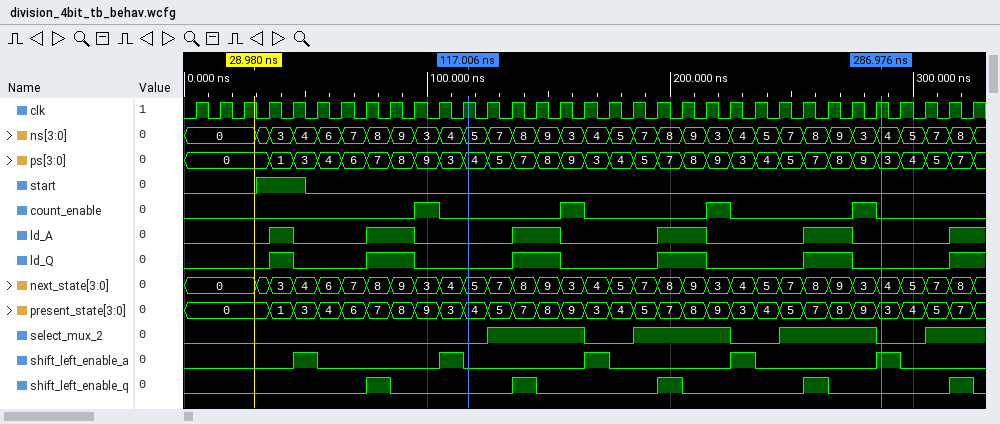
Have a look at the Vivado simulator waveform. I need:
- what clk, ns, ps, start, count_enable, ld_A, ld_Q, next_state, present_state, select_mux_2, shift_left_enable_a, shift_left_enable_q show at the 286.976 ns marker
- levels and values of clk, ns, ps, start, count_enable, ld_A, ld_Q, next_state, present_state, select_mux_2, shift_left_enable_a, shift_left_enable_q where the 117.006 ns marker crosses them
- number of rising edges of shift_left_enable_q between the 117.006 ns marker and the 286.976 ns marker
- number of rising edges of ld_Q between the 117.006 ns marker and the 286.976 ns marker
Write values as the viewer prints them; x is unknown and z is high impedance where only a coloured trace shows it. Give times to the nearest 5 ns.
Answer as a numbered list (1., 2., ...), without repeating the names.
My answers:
1. clk=1, ns=4, ps=3, start=0, count_enable=0, ld_A=0, ld_Q=0, next_state=4, present_state=3, select_mux_2=0, shift_left_enable_a=1, shift_left_enable_q=0
2. clk=1, ns=5, ps=4, start=0, count_enable=0, ld_A=0, ld_Q=0, next_state=5, present_state=4, select_mux_2=0, shift_left_enable_a=0, shift_left_enable_q=0
3. 3
4. 3
